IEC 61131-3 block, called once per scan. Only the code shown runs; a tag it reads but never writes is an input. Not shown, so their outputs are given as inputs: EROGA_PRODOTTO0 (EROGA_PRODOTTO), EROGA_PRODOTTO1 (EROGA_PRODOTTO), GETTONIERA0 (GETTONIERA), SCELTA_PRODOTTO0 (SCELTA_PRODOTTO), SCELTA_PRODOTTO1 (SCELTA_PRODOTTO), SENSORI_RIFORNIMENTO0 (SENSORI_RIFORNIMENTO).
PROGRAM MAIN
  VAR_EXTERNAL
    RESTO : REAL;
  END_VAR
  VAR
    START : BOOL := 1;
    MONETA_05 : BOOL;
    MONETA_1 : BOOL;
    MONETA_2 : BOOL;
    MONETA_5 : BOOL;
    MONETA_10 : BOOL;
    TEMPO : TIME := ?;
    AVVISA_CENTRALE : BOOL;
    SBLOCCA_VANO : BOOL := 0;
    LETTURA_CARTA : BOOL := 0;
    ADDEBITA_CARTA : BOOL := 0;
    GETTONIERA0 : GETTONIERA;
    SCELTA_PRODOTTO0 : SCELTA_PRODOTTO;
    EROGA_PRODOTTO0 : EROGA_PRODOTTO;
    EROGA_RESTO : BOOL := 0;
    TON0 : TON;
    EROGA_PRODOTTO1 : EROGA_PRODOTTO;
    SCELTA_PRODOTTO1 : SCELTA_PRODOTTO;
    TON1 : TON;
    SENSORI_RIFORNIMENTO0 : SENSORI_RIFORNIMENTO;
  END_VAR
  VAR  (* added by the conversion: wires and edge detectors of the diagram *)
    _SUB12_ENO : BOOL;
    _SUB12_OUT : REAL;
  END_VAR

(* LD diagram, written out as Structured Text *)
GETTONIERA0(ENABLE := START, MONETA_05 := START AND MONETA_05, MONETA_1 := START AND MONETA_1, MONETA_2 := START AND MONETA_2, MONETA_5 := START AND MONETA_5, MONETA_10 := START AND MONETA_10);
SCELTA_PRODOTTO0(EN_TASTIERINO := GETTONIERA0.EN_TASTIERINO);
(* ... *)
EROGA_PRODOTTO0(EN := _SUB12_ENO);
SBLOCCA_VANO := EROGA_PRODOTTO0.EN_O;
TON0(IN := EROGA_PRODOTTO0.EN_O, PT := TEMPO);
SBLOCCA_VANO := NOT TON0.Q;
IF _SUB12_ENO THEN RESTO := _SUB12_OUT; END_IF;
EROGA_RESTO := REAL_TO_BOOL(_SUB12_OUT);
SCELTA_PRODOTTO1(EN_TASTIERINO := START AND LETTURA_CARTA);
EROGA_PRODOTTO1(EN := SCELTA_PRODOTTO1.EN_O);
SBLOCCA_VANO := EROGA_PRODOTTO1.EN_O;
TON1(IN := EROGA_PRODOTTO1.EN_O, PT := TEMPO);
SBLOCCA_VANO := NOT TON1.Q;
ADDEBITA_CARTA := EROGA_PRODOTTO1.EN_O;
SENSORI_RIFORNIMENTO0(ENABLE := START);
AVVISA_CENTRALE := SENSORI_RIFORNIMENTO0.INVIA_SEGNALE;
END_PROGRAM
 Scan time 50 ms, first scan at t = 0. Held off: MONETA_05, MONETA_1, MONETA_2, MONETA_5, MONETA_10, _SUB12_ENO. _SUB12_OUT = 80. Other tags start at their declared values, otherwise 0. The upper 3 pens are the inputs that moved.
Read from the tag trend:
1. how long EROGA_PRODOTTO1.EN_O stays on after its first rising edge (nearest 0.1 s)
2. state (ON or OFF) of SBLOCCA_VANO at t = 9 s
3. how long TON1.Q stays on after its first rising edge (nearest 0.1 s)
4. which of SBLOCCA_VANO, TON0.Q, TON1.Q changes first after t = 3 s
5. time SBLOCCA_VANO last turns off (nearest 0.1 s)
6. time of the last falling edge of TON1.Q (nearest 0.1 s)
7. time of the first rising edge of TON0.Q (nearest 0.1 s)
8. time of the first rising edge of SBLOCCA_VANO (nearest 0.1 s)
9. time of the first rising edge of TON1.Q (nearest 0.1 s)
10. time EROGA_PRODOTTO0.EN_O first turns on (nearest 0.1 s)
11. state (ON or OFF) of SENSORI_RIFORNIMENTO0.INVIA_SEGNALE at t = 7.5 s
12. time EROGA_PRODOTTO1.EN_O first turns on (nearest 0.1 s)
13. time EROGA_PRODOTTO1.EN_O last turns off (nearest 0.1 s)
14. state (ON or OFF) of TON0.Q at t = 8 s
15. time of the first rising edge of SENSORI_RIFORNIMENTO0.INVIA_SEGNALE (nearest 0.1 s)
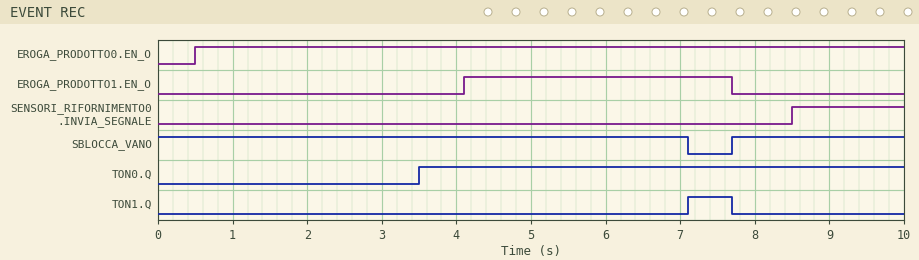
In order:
3.6 s
ON
0.6 s
TON0.Q
7.1 s
7.7 s
3.5 s
7.7 s
7.1 s
0.5 s
OFF
4.1 s
7.7 s
ON
8.5 s
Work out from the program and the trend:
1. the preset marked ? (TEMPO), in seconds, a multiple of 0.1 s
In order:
3.0 s
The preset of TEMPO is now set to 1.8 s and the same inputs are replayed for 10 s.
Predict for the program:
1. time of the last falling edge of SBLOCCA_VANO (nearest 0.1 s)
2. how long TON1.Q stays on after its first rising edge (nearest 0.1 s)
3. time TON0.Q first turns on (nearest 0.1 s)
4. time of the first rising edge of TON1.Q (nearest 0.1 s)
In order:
5.9 s
1.8 s
2.3 s
5.9 s
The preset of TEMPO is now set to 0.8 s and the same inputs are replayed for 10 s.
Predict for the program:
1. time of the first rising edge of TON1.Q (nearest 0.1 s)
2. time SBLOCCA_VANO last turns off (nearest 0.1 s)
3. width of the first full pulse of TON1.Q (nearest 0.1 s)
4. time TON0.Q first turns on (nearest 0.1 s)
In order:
4.9 s
4.9 s
2.8 s
1.3 s
